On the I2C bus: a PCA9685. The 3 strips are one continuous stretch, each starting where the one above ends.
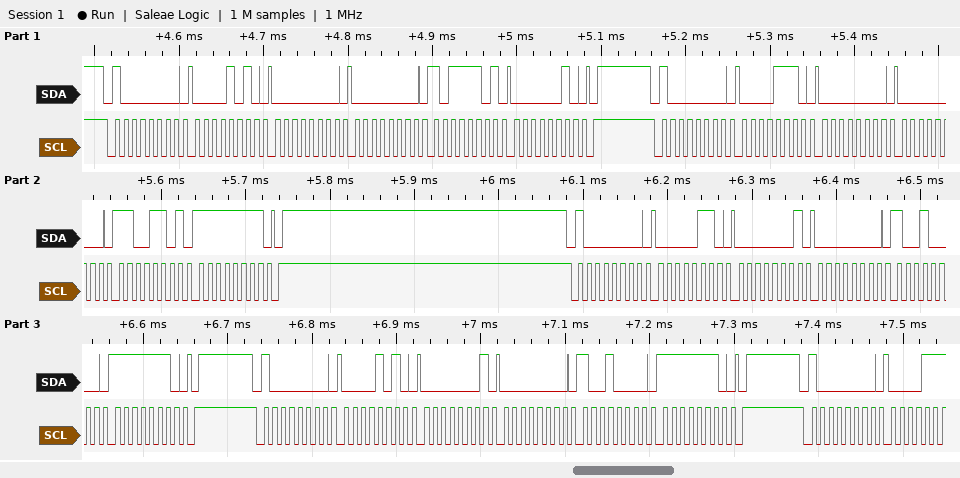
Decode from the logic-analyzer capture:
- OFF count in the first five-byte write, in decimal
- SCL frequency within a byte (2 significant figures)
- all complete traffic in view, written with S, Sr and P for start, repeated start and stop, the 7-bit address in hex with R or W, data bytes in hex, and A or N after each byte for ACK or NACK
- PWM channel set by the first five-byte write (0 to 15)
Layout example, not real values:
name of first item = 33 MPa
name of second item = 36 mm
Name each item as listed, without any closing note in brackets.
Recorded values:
OFF count in the first five-byte write, in decimal = 701
SCL frequency within a byte = 100 kHz
all complete traffic in view, written with S, Sr and P for start, repeated start and stop, the 7-bit address in hex with R or W, data bytes in hex, and A or N after each byte for ACK or NACK = S 40W A 0A A 00 A 00 A BD A 02 A P S 40W A 0E A 00 A 00 A CD A FF A P S 40W A 06 A 01 A 00 A 90 A FE A P S 40W A 0A A 01 A 00 A 90 A FE A P S 40W A
PWM channel set by the first five-byte write = 1
